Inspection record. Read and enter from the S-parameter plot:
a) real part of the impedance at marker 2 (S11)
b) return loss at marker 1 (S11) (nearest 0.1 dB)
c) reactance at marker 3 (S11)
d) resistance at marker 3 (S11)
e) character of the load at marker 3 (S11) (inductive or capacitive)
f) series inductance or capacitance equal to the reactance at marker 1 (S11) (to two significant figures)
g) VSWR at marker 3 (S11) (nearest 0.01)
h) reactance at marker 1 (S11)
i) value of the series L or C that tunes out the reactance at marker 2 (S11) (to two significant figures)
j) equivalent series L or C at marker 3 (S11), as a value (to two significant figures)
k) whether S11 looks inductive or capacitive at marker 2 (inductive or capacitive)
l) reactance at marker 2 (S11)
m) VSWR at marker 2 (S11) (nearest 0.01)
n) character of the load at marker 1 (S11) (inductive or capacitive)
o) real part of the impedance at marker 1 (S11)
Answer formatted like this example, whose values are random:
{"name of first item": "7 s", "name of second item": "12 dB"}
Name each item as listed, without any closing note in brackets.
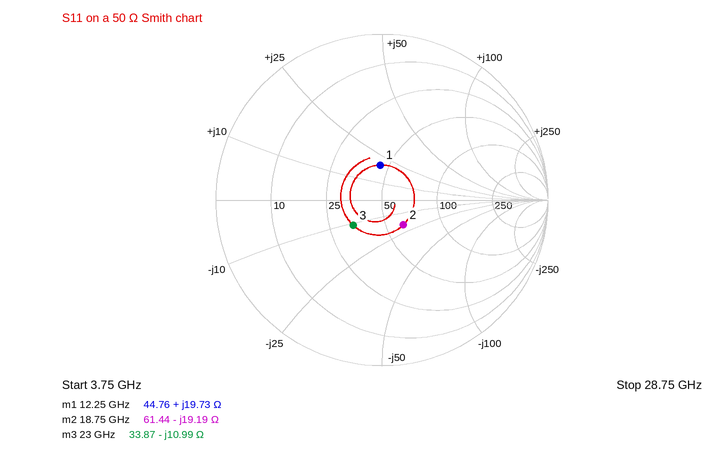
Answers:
{"real part of the impedance at marker 2": "61.44 Ω", "return loss at marker 1 (S11)": "13.5 dB", "reactance at marker 3": "-10.99 Ω", "resistance at marker 3": "33.87 Ω", "character of the load at marker 3 (S11)": "capacitive", "series inductance or capacitance equal to the reactance at marker 1 (S11)": "260 pH", "VSWR at marker 3 (S11)": "1.60", "reactance at marker 1": "+19.73 Ω", "value of the series L or C that tunes out the reactance at marker 2 (S11)": "160 pH", "equivalent series L or C at marker 3 (S11), as a value": "630 fF", "whether S11 looks inductive or capacitive at marker 2": "capacitive", "reactance at marker 2": "-19.19 Ω", "VSWR at marker 2 (S11)": "1.49", "character of the load at marker 1 (S11)": "inductive", "real part of the impedance at marker 1": "44.76 Ω"}
